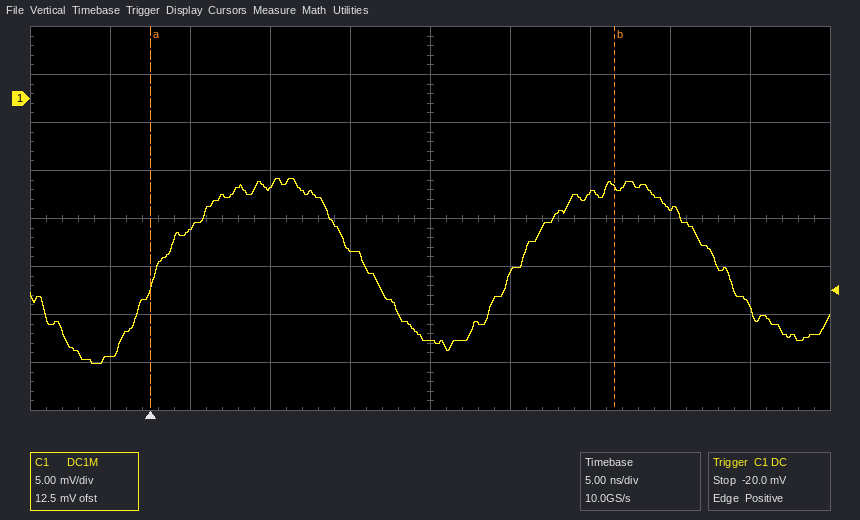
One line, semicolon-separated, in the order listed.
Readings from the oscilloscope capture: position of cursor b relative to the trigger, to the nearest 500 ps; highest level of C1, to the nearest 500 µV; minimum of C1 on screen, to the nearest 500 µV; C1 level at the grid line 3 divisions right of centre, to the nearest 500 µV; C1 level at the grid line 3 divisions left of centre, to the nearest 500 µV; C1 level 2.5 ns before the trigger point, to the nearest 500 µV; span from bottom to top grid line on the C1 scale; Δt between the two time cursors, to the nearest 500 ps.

+29.0 ns; -8.5 mV; -27.5 mV; -11.5 mV; -13.5 mV; -27.0 mV; 40 mV; 29.0 ns
